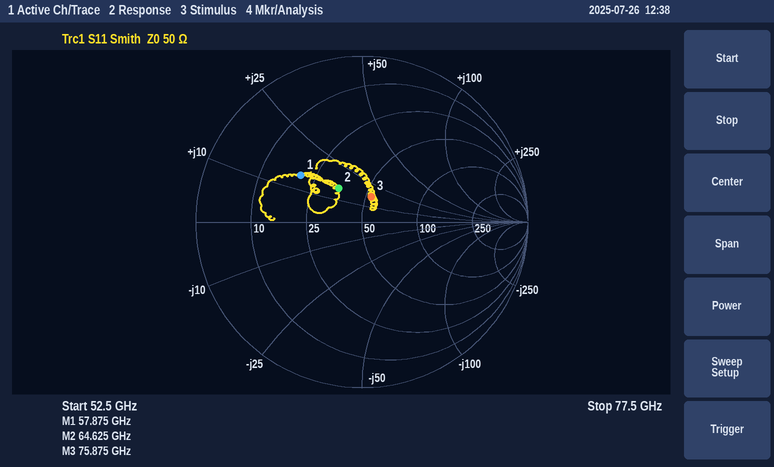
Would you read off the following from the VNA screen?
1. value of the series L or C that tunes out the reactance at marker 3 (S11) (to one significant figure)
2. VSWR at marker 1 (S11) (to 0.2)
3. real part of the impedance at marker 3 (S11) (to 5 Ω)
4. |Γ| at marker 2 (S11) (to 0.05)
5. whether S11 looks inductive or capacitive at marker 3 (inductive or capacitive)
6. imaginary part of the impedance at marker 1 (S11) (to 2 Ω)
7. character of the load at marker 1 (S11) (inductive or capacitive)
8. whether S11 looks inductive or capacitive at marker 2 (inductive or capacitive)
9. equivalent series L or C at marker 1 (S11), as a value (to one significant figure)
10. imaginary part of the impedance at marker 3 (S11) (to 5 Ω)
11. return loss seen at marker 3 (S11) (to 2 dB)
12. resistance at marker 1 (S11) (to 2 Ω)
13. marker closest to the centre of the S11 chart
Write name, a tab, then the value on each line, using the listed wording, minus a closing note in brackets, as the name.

value of the series L or C that tunes out the reactance at marker 3 (S11)	100 fF
VSWR at marker 1 (S11)	2.8
real part of the impedance at marker 3 (S11)	55 Ω
|Γ| at marker 2 (S11)	0.25
whether S11 looks inductive or capacitive at marker 3	inductive
imaginary part of the impedance at marker 1 (S11)	+14 Ω
character of the load at marker 1 (S11)	inductive
whether S11 looks inductive or capacitive at marker 2	inductive
equivalent series L or C at marker 1 (S11), as a value	40 pH
imaginary part of the impedance at marker 3 (S11)	+15 Ω
return loss seen at marker 3 (S11)	16 dB
resistance at marker 1 (S11)	20 Ω
marker closest to the centre of the S11 chart	marker 3
